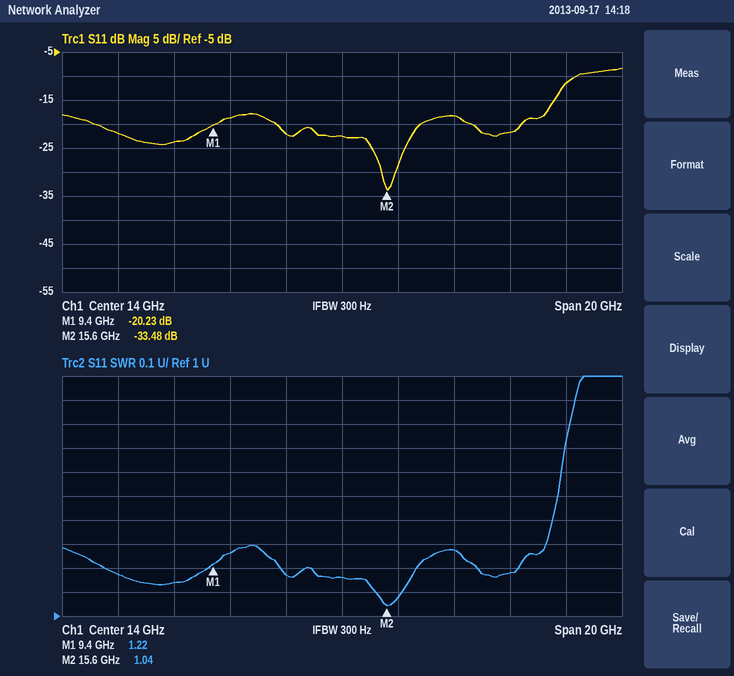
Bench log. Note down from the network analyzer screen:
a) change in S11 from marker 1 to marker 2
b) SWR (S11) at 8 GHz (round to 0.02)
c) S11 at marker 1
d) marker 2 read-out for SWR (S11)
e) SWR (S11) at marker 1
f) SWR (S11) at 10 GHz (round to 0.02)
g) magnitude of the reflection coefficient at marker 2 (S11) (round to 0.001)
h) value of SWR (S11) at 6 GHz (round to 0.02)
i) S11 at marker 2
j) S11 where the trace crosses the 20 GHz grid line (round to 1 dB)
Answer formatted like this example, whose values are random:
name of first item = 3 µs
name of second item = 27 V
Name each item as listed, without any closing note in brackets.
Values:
change in S11 from marker 1 to marker 2 = -13.25 dB
SWR (S11) at 8 GHz = 1.14
S11 at marker 1 = -20.23 dB
marker 2 read-out for SWR = 1.04
SWR (S11) at marker 1 = 1.22
SWR (S11) at 10 GHz = 1.26
magnitude of the reflection coefficient at marker 2 (S11) = 0.021
value of SWR (S11) at 6 GHz = 1.18
S11 at marker 2 = -33.48 dB
S11 where the trace crosses the 20 GHz grid line = -22 dB
